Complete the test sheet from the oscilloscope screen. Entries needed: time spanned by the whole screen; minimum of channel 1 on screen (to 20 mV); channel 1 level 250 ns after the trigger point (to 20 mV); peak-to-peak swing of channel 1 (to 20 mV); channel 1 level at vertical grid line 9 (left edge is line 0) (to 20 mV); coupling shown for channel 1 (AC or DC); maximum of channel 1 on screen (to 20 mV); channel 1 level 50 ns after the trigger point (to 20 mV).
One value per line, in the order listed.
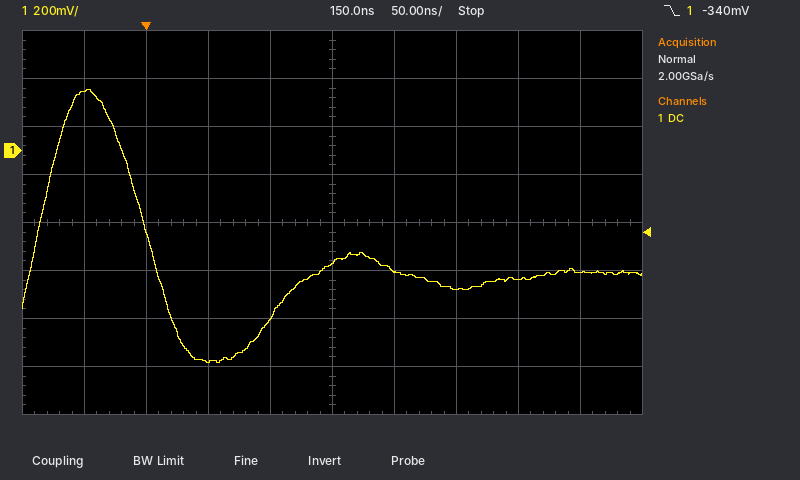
500 ns
-880 mV
-580 mV
1.14 V
-500 mV
DC
260 mV
-880 mV
